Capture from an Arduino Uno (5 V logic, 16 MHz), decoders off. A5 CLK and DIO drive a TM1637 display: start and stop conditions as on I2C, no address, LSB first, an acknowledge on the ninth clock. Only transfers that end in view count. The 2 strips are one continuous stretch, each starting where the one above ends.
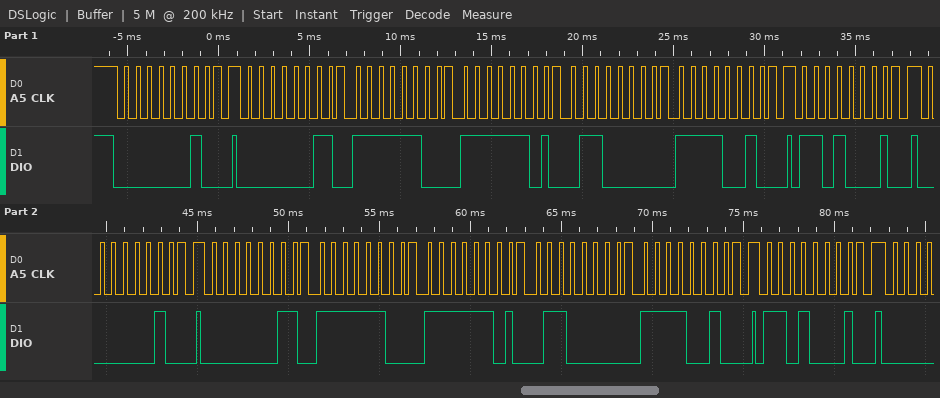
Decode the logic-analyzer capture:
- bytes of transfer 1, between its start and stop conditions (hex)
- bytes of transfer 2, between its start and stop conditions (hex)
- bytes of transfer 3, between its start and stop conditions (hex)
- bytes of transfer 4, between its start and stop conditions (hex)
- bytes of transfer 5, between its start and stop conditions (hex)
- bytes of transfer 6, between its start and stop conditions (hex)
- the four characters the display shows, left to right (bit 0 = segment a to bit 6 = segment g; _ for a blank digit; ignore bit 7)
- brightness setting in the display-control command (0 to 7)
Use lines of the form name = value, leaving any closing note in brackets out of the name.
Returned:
bytes of transfer 1, between its start and stop conditions = 40
bytes of transfer 2, between its start and stop conditions = C0 3F BF 06 4F
bytes of transfer 3, between its start and stop conditions = 8B
bytes of transfer 4, between its start and stop conditions = 40
bytes of transfer 5, between its start and stop conditions = C0 3F BF 06 4F
bytes of transfer 6, between its start and stop conditions = 8B
the four characters the display shows, left to right = 0013
brightness setting in the display-control command = 3
